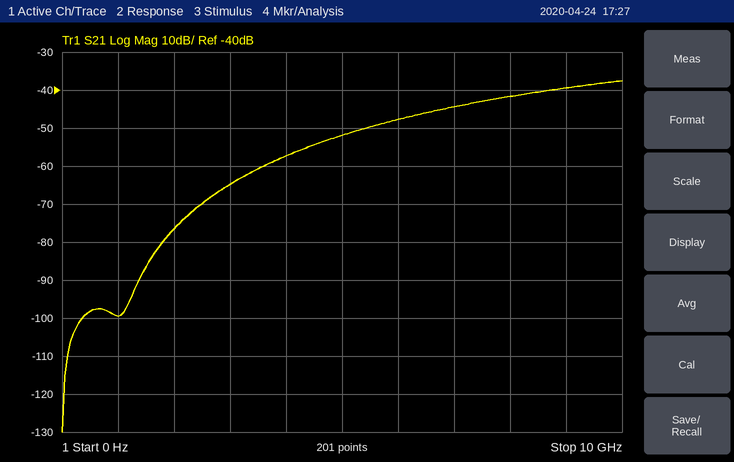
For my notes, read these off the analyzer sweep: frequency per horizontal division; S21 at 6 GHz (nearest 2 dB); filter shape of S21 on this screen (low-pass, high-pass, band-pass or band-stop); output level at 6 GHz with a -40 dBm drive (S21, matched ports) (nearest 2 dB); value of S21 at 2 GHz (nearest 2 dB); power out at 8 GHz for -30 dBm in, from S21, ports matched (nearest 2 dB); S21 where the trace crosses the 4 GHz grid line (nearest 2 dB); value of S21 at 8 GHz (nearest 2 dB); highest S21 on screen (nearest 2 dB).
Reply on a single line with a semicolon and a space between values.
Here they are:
1 GHz; -48 dB; high-pass; -88 dBm; -76 dB; -72 dBm; -58 dB; -42 dB; -38 dB
